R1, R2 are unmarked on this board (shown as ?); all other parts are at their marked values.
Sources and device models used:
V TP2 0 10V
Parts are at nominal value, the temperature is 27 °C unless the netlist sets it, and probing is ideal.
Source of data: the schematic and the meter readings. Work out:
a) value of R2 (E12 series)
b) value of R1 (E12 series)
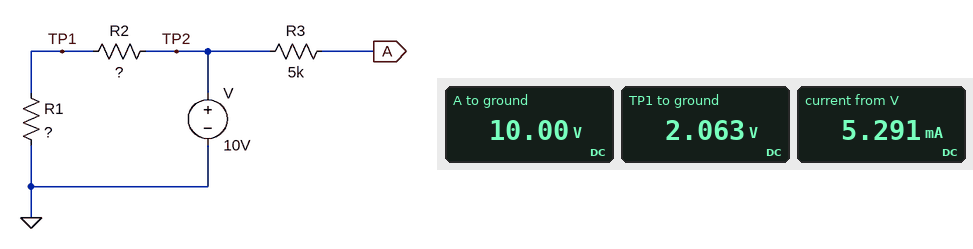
1.5 kΩ
390 Ω
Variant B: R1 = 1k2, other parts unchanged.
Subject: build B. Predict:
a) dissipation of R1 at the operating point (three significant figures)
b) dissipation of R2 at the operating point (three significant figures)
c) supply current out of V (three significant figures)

16.5 mW
20.6 mW
3.70 mA
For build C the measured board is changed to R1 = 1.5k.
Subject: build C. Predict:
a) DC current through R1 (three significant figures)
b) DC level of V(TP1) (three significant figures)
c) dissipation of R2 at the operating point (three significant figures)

3.33 mA
5.00 V
16.7 mW
